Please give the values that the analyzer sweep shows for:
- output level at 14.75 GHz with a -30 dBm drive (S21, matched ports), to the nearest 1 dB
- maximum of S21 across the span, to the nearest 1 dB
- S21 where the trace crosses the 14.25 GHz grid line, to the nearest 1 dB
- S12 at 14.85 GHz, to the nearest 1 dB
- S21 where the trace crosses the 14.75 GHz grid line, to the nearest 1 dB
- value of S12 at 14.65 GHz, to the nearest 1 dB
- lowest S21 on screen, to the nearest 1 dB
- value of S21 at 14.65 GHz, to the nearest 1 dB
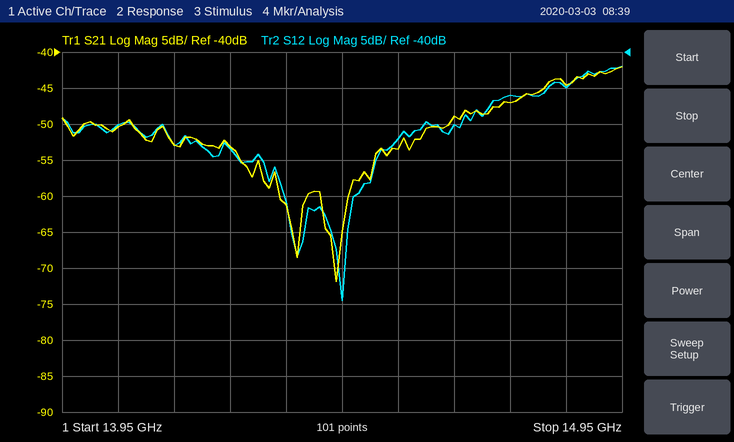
-77 dBm
-42 dB
-53 dB
-45 dB
-47 dB
-50 dB
-72 dB
-49 dB
